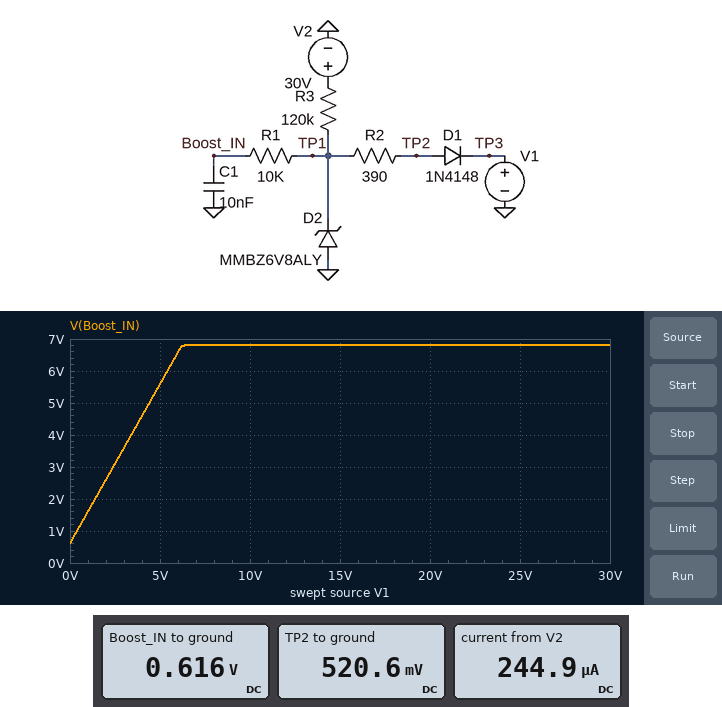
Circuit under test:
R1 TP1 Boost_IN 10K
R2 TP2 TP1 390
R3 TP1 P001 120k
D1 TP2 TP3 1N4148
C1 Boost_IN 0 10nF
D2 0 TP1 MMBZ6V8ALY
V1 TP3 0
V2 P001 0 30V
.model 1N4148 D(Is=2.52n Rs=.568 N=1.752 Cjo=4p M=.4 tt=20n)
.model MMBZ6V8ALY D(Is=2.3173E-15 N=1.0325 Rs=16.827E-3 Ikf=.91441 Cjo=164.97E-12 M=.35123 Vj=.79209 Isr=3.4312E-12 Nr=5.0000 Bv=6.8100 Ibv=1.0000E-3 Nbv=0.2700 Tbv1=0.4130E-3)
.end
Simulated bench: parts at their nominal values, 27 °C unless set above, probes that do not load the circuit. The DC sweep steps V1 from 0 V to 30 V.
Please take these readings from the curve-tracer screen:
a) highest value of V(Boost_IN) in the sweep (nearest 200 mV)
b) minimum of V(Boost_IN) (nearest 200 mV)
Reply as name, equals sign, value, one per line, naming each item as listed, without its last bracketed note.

highest value of V(Boost_IN) in the sweep = 6.8 V
minimum of V(Boost_IN) = 600 mV
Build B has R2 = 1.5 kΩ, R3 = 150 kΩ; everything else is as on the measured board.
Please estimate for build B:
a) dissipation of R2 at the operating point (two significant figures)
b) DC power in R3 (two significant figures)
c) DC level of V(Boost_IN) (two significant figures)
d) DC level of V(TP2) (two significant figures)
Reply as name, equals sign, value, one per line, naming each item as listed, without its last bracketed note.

dissipation of R2 at the operating point = 57 µW
DC power in R3 = 5.7 mW
DC level of V(Boost_IN) = 800 mV
DC level of V(TP2) = 510 mV
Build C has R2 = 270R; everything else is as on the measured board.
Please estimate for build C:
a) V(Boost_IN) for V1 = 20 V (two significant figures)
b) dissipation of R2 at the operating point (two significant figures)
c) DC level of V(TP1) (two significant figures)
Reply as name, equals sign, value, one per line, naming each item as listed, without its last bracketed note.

V(Boost_IN) for V1 = 20 V = 6.8 V
dissipation of R2 at the operating point = 16 µW
DC level of V(TP1) = 590 mV
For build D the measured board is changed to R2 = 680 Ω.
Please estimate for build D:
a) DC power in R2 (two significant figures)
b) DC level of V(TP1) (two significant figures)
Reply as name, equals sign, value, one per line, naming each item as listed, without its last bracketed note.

DC power in R2 = 41 µW
DC level of V(TP1) = 690 mV
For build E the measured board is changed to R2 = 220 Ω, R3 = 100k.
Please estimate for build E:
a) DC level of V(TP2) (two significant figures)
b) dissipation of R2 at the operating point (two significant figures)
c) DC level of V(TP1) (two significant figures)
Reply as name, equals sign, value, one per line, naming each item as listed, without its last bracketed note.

DC level of V(TP2) = 530 mV
dissipation of R2 at the operating point = 19 µW
DC level of V(TP1) = 590 mV
